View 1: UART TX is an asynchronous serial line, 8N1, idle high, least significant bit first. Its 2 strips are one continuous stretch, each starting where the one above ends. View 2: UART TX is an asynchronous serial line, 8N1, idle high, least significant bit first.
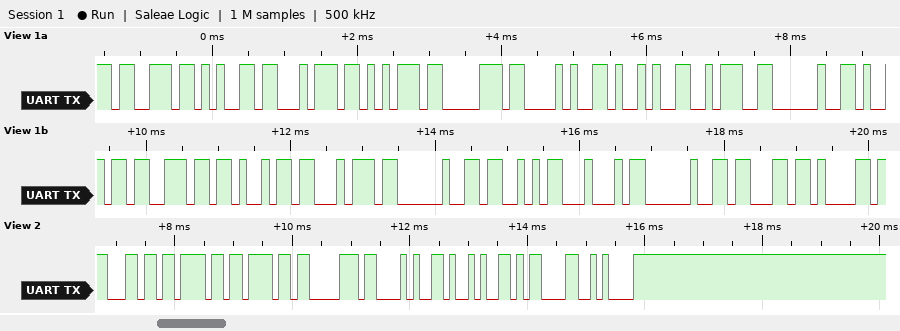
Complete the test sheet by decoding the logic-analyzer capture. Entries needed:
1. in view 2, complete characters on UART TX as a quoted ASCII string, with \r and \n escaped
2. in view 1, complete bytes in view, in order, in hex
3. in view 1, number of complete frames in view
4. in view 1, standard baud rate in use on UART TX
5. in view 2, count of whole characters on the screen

"loop()\r\n"
73 65 74 75 70 28 29 3A 20 69 6E 69 74 20 53 44 20 63 61
19
9600 baud
8
